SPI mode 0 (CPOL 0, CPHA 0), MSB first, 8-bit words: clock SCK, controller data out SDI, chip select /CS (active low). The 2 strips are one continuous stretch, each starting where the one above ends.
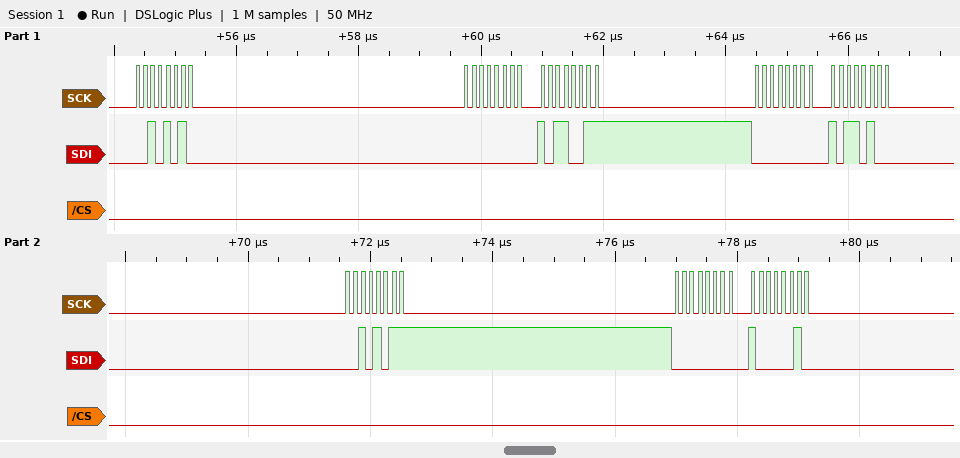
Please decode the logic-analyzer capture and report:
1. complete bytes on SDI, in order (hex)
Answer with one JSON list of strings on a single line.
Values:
["2A 00 B3 00 B4 2B 00 82"]
